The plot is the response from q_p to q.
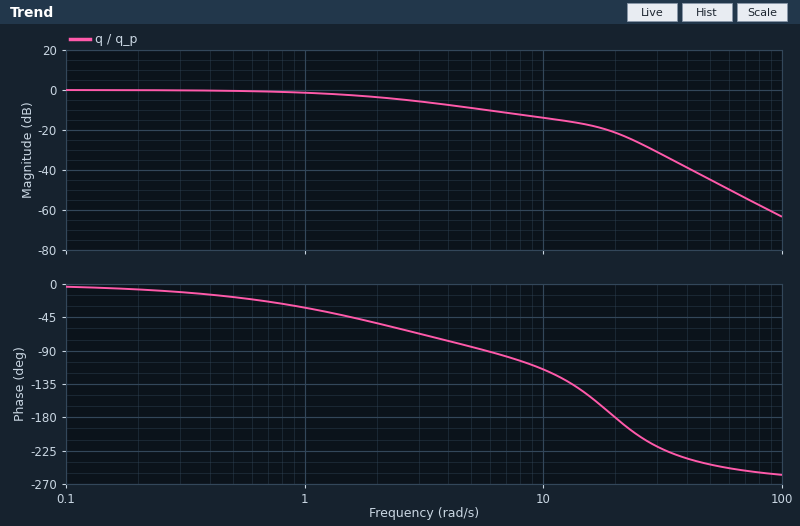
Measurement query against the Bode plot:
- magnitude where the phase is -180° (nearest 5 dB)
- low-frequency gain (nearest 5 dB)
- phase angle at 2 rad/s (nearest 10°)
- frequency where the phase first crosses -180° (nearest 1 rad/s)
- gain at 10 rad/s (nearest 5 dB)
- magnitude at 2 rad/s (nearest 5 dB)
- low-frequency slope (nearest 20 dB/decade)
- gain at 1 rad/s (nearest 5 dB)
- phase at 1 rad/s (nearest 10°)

-20 dB
0 dB
-50°
20 rad/s
-15 dB
-5 dB
0 dB/decade
0 dB
-30°
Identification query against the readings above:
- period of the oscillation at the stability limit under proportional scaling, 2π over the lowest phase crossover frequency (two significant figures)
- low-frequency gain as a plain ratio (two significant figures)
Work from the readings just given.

0.31 s
1.0
